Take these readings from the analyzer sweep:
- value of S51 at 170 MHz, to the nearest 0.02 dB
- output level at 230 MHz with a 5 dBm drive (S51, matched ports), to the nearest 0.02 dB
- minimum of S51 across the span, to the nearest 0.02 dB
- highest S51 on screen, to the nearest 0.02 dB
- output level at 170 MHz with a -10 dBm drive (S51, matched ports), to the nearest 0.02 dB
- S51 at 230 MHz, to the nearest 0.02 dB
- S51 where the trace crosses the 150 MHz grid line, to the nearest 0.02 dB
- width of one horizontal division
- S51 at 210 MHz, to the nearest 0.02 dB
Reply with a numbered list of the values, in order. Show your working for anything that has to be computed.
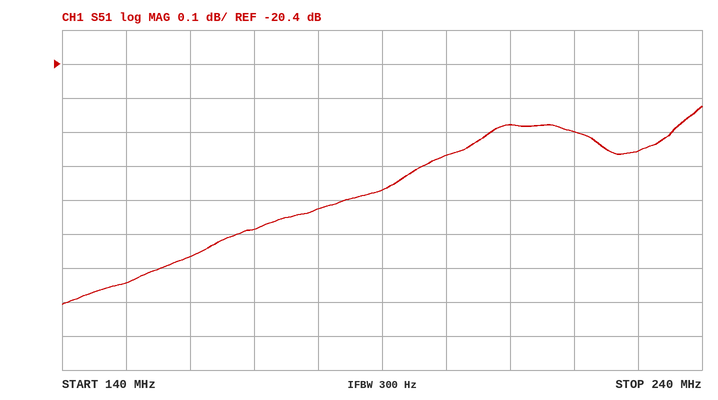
1. -20.88 dB
2. 5 dBm + (-20.66 dB) = -15.66 dBm
3. -21.10 dB
4. -20.52 dB
5. -10 dBm + (-20.88 dB) = -30.88 dBm
6. -20.66 dB
7. -21.04 dB
8. 10 MHz
9. -20.58 dB
